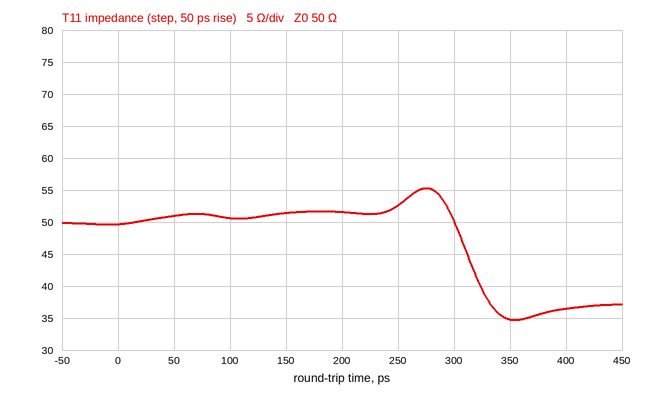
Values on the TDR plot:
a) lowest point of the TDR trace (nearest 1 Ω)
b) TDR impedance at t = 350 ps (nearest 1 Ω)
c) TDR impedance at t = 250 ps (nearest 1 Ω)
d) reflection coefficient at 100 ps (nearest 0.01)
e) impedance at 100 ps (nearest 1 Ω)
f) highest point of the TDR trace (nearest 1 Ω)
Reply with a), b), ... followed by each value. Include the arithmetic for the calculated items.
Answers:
a) 35 Ω
b) 35 Ω
c) 53 Ω
d) (51 − 50)/(51 + 50) ≈ +0.01
e) 51 Ω
f) 55 Ω
